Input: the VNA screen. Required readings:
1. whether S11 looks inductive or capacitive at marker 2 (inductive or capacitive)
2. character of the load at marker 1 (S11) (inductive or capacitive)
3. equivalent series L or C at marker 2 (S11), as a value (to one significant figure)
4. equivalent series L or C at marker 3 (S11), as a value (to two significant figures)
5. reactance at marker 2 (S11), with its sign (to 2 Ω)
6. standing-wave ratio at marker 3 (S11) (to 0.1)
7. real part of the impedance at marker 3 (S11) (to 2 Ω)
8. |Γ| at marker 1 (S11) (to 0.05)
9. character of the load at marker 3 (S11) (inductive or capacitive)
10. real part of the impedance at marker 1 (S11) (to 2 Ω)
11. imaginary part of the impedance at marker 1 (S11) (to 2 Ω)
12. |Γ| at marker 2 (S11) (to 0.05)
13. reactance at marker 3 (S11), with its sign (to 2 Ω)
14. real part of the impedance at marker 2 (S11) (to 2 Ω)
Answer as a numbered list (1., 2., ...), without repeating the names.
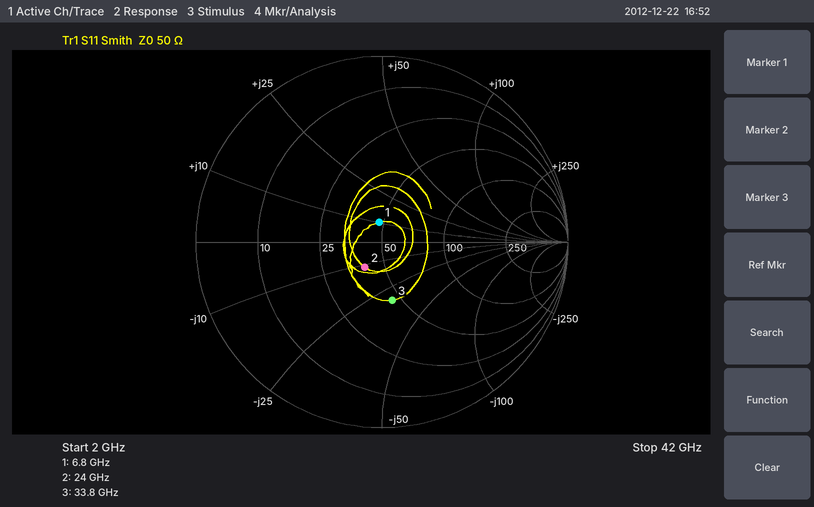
1. capacitive
2. inductive
3. 600 fF
4. 150 fF
5. -12 Ω
6. 1.9
7. 46 Ω
8. 0.10
9. capacitive
10. 48 Ω
11. +10 Ω
12. 0.15
13. -32 Ω
14. 40 Ω
